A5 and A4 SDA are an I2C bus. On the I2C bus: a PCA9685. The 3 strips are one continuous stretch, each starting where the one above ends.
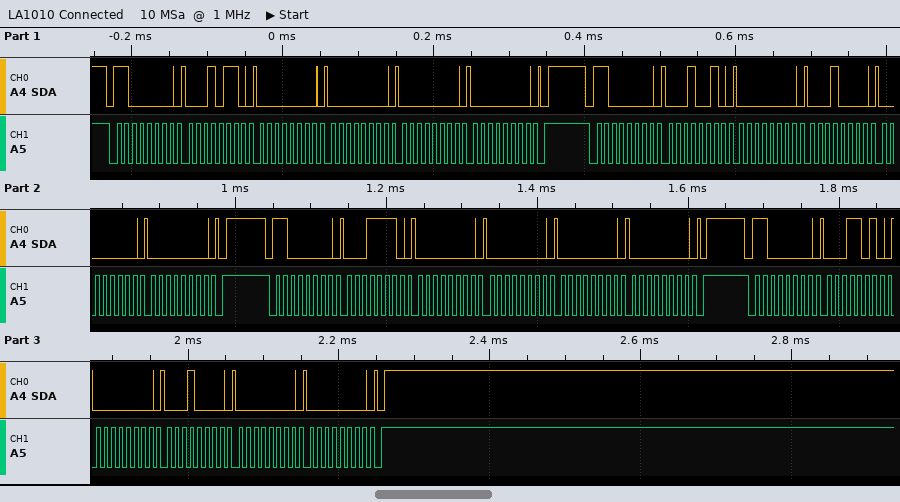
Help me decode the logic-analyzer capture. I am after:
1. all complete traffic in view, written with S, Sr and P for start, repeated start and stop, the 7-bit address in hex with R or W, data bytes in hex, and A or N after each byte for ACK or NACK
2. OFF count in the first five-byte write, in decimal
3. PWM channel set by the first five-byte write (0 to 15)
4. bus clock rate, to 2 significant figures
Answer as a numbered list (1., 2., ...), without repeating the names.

1. S 60W A 16 A 00 A 00 A 00 A 00 A P S 60W A 12 A 00 A 10 A 00 A 00 A P S 60W A 1E A 00 A 00 A 00 A 00 A P S 60W A 1A A 00 A 10 A 00 A 00 A P
2. 0
3. 4
4. 100 kHz
